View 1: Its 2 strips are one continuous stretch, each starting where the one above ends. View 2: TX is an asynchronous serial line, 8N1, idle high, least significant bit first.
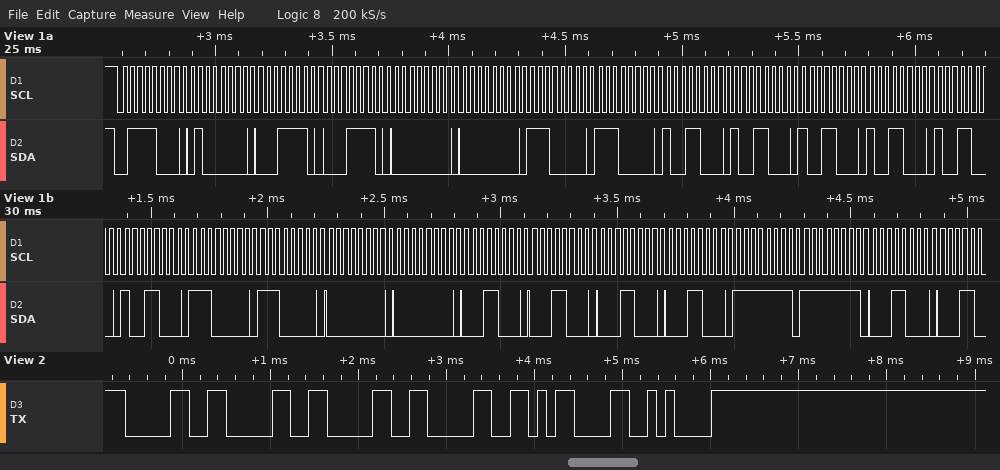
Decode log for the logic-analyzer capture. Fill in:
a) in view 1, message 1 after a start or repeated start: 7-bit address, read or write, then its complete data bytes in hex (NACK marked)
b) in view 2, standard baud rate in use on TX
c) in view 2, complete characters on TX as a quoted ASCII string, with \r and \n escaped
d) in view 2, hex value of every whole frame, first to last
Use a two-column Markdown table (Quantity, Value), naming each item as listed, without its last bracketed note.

| Quantity | Value |
|---|---|
| in view 1, message 1 after a start or repeated start: 7-bit address, read or write, then its complete data bytes in hex | 0x3C write: 40 1E 1E 00 00 E0 E0 98 98 98 98 98 98 E0 E0 00 00 18 18 18 18 FF FF 18 |
| in view 2, standard baud rate in use on TX | 9600 baud |
| in view 2, complete characters on TX as a quoted ASCII string, with \r and \n escaped | "0000\r\n" |
| in view 2, hex value of every whole frame, first to last | 30 30 30 30 0D 0A |
